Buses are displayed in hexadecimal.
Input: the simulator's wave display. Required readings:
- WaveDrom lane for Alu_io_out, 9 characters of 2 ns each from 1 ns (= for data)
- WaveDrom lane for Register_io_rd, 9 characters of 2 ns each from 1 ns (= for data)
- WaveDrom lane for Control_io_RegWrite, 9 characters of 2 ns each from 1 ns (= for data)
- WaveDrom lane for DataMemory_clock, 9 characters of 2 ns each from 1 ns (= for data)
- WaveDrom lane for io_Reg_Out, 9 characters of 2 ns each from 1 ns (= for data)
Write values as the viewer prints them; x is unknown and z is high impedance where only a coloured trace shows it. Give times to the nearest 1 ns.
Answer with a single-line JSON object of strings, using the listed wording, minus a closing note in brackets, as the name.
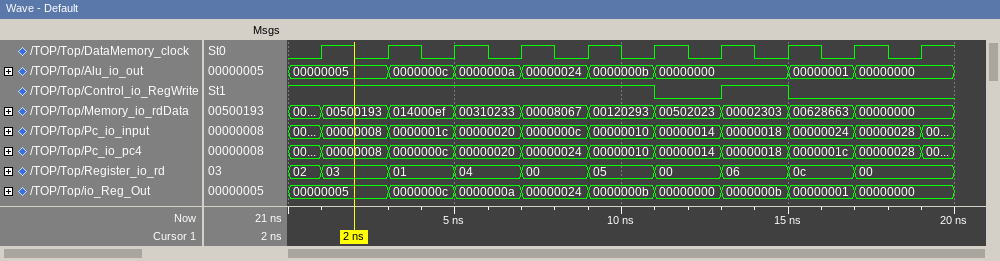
{"WaveDrom lane for Alu_io_out, 9 characters of 2 ns each from 1 ns": "{name: 'Alu_io_out', wave: '======.==', data: '00000005 0000000c 0000000a 00000024 0000000b 00000000 00000001 00000000'}", "WaveDrom lane for Register_io_rd, 9 characters of 2 ns each from 1 ns": "{name: 'Register_io_rd', wave: '=========', data: '03 01 04 00 05 00 06 0c 00'}", "WaveDrom lane for Control_io_RegWrite, 9 characters of 2 ns each from 1 ns": "{name: 'Control_io_RegWrite', wave: '1....010.'}", "WaveDrom lane for DataMemory_clock, 9 characters of 2 ns each from 1 ns": "{name: 'DataMemory_clock', wave: 'p........'}", "WaveDrom lane for io_Reg_Out, 9 characters of 2 ns each from 1 ns": "{name: 'io_Reg_Out', wave: '=========', data: '00000005 0000000c 0000000a 00000024 0000000b 00000000 0000000b 00000001 00000000'}"}
